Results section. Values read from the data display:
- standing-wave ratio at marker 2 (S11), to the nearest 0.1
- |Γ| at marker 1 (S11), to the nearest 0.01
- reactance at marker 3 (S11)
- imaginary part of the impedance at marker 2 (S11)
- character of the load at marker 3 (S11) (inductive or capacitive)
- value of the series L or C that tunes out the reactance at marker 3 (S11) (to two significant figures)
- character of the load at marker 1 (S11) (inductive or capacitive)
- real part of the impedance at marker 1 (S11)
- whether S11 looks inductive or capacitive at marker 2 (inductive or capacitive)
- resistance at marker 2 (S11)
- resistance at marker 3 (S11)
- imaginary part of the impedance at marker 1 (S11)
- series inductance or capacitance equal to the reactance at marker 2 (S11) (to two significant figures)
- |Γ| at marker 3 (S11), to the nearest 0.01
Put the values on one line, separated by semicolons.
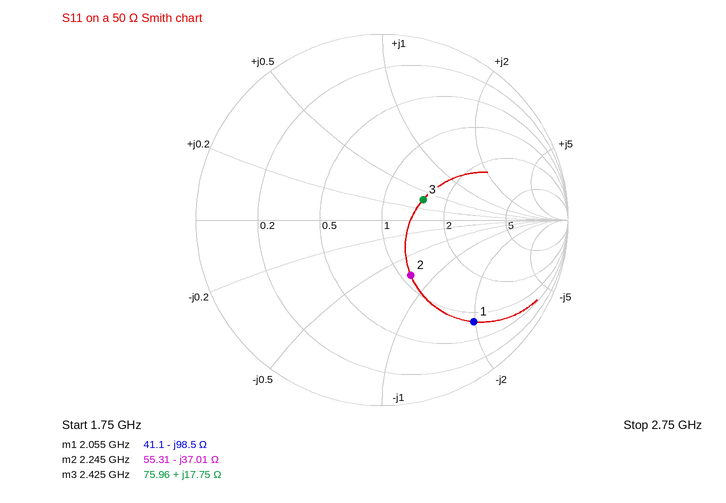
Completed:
2.0; 0.74; +17.75 Ω; -37.01 Ω; inductive; 3.7 pF; capacitive; 41.1 Ω; capacitive; 55.31 Ω; 75.96 Ω; -98.5 Ω; 1.9 pF; 0.25
